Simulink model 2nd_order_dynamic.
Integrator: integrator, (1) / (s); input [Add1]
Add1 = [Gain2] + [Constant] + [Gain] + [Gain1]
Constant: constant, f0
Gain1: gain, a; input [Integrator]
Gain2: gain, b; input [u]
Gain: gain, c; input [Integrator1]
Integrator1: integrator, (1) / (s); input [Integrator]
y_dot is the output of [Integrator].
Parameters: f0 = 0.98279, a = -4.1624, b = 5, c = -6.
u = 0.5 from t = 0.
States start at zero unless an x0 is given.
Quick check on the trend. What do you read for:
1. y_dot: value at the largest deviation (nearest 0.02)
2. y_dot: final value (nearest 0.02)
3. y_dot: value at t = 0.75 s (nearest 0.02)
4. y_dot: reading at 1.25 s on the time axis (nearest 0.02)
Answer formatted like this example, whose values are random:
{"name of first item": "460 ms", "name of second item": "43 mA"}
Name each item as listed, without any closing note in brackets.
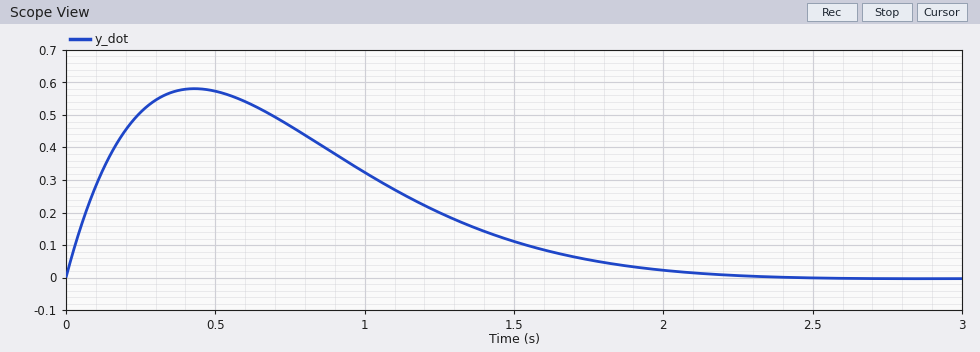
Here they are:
{"y_dot: value at the largest deviation": "0.58", "y_dot: final value": "0.00", "y_dot: value at t = 0.75 s": "0.46", "y_dot: reading at 1.25 s on the time axis": "0.20"}
